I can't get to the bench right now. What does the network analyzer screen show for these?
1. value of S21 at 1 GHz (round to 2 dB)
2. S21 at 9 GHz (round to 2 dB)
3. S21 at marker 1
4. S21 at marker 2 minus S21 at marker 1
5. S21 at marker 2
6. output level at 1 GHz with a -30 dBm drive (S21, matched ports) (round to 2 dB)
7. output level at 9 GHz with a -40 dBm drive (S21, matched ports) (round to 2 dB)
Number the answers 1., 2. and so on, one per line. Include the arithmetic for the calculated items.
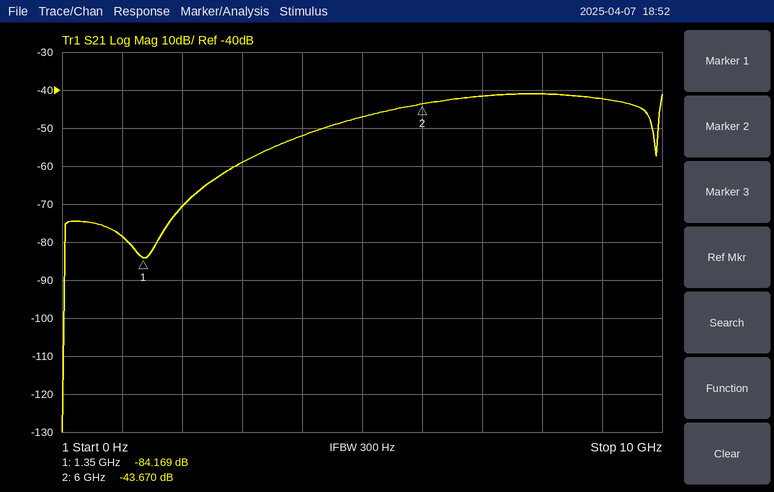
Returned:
1. -78 dB
2. -42 dB
3. -84.169 dB
4. -43.67 − (-84.169) = 40.499 dB
5. -43.670 dB
6. -30 dBm + (-78 dB) = -108 dBm
7. -40 dBm + (-42 dB) = -82 dBm
